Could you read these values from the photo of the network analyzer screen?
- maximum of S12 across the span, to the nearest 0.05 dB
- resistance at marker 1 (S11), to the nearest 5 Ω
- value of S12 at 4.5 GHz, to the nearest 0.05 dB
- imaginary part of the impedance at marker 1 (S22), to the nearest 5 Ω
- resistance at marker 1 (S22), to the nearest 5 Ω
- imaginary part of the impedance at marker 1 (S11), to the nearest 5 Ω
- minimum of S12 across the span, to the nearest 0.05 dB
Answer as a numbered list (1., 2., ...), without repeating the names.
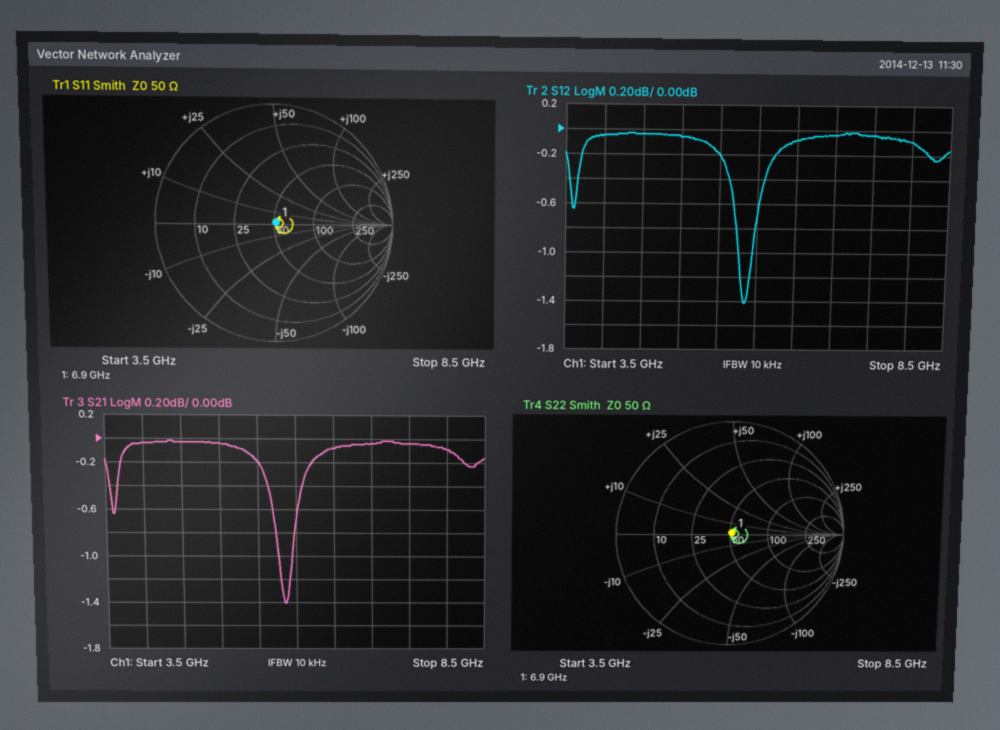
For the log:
1. 0.00 dB
2. 50 Ω
3. -0.05 dB
4. 0 Ω
5. 50 Ω
6. 0 Ω
7. -1.40 dB
